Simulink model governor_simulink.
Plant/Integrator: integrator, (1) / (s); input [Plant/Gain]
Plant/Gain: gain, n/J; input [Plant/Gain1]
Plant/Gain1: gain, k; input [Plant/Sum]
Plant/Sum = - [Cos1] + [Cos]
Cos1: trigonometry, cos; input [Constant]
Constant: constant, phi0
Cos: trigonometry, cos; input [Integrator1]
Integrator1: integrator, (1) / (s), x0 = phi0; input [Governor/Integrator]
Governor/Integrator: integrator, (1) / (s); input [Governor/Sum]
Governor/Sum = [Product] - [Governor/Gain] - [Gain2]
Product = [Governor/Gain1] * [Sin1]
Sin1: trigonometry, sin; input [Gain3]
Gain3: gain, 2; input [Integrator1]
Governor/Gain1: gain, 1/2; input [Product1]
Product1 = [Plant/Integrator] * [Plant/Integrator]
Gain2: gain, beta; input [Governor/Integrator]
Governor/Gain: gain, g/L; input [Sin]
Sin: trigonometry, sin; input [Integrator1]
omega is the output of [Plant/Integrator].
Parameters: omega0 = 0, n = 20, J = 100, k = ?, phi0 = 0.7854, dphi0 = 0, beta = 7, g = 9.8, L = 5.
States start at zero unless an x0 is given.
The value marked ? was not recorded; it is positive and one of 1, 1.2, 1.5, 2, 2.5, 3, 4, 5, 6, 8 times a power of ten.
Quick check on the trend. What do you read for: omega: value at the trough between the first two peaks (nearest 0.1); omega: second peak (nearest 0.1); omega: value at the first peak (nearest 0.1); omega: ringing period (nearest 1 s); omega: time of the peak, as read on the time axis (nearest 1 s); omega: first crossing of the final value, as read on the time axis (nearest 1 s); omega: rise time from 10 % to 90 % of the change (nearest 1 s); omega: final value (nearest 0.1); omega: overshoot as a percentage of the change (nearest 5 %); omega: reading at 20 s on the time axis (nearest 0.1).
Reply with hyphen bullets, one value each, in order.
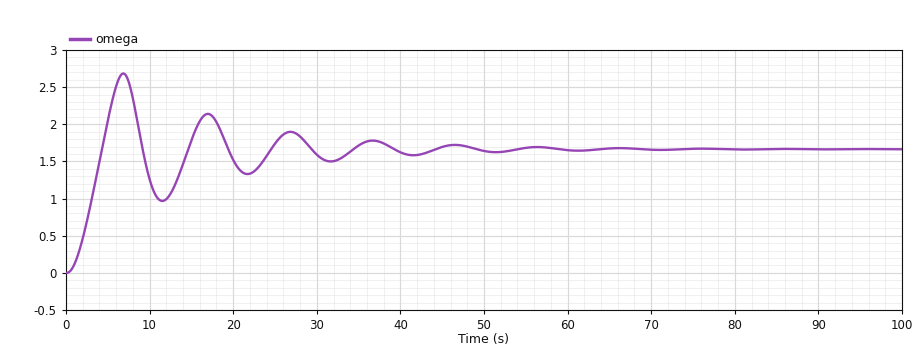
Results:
- 1.0
- 2.1
- 2.7
- 10 s
- 7 s
- 4 s
- 3 s
- 1.7
- 60 %
- 1.5
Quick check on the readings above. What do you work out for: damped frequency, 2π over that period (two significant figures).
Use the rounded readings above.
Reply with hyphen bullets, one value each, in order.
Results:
- 0.63 rad/s
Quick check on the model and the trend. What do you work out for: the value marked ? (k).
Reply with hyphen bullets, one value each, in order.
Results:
- 12
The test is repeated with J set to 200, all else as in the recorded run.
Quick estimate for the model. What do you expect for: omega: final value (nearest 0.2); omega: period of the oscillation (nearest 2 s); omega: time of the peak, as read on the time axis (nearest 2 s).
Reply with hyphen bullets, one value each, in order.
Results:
- 1.6
- 14 s
- 10 s
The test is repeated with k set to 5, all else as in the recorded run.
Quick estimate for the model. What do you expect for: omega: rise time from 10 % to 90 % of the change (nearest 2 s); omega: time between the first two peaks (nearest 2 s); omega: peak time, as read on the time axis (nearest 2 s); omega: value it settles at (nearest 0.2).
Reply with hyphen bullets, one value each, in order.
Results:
- 6 s
- 16 s
- 12 s
- 1.6
